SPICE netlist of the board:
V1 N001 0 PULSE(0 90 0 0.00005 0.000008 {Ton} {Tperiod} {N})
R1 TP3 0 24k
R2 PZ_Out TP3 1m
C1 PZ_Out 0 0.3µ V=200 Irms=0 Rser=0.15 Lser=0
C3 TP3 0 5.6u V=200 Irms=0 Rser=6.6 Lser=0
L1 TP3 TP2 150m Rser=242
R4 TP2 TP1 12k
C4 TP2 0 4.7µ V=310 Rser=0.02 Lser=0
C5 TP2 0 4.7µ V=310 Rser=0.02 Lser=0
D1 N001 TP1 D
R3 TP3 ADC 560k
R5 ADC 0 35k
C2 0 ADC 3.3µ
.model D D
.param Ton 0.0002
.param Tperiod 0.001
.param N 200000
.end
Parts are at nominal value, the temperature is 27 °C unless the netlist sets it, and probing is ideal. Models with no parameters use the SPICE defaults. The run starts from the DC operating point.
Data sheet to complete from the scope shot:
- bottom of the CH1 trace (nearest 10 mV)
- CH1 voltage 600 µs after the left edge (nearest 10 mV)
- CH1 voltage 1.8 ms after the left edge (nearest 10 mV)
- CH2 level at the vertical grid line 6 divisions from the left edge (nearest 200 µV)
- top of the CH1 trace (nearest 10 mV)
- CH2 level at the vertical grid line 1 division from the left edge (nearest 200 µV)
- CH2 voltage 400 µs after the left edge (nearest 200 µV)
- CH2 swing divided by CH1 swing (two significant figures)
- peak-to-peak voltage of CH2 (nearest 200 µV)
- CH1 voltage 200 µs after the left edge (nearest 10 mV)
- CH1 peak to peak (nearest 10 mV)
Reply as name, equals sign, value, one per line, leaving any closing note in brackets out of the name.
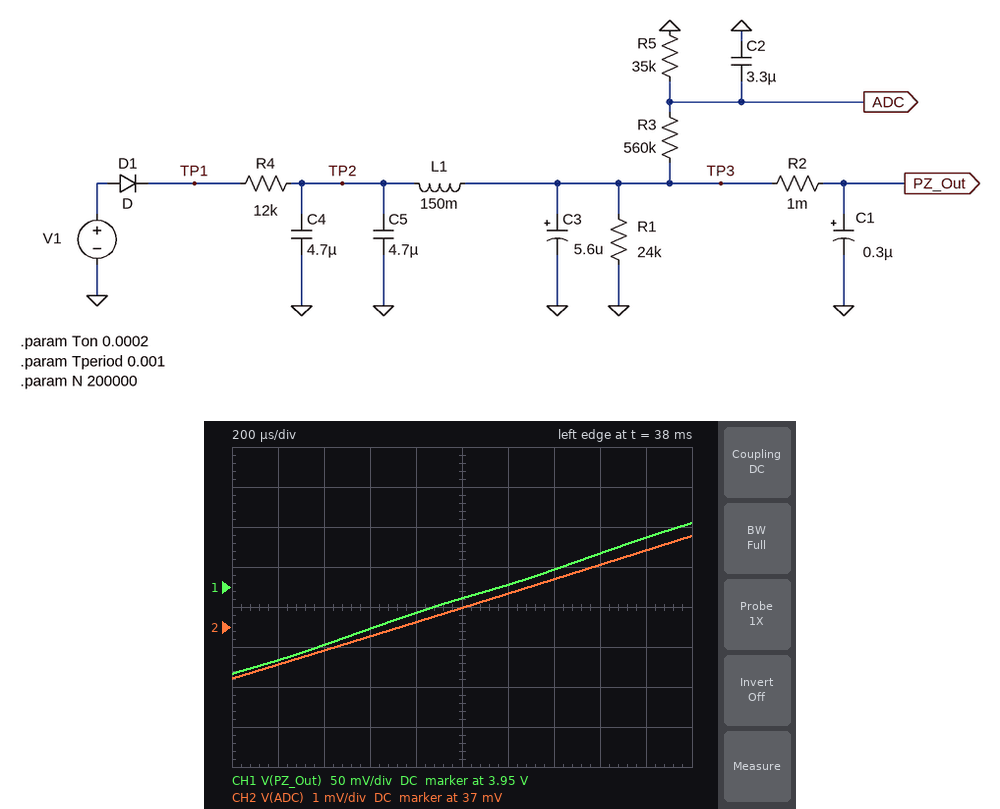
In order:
bottom of the CH1 trace = 3.84 V
CH1 voltage 600 µs after the left edge = 3.90 V
CH1 voltage 1.8 ms after the left edge = 4.01 V
CH2 level at the vertical grid line 6 divisions from the left edge = 37.8 mV
top of the CH1 trace = 4.03 V
CH2 level at the vertical grid line 1 division from the left edge = 36.0 mV
CH2 voltage 400 µs after the left edge = 36.4 mV
CH2 swing divided by CH1 swing = 0.019
peak-to-peak voltage of CH2 = 3.6 mV
CH1 voltage 200 µs after the left edge = 3.86 V
CH1 peak to peak = 190 mV
